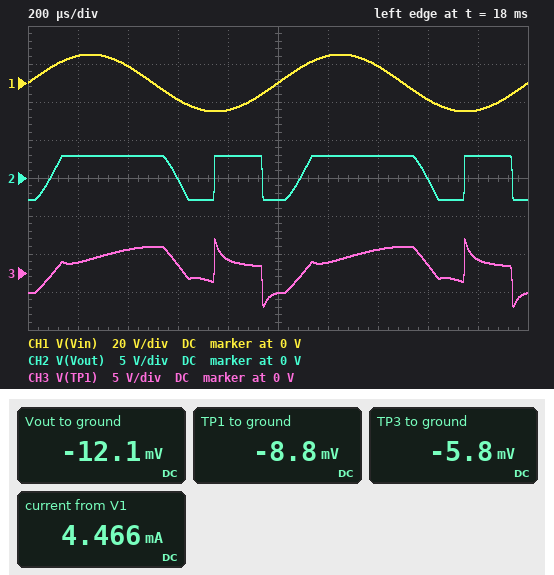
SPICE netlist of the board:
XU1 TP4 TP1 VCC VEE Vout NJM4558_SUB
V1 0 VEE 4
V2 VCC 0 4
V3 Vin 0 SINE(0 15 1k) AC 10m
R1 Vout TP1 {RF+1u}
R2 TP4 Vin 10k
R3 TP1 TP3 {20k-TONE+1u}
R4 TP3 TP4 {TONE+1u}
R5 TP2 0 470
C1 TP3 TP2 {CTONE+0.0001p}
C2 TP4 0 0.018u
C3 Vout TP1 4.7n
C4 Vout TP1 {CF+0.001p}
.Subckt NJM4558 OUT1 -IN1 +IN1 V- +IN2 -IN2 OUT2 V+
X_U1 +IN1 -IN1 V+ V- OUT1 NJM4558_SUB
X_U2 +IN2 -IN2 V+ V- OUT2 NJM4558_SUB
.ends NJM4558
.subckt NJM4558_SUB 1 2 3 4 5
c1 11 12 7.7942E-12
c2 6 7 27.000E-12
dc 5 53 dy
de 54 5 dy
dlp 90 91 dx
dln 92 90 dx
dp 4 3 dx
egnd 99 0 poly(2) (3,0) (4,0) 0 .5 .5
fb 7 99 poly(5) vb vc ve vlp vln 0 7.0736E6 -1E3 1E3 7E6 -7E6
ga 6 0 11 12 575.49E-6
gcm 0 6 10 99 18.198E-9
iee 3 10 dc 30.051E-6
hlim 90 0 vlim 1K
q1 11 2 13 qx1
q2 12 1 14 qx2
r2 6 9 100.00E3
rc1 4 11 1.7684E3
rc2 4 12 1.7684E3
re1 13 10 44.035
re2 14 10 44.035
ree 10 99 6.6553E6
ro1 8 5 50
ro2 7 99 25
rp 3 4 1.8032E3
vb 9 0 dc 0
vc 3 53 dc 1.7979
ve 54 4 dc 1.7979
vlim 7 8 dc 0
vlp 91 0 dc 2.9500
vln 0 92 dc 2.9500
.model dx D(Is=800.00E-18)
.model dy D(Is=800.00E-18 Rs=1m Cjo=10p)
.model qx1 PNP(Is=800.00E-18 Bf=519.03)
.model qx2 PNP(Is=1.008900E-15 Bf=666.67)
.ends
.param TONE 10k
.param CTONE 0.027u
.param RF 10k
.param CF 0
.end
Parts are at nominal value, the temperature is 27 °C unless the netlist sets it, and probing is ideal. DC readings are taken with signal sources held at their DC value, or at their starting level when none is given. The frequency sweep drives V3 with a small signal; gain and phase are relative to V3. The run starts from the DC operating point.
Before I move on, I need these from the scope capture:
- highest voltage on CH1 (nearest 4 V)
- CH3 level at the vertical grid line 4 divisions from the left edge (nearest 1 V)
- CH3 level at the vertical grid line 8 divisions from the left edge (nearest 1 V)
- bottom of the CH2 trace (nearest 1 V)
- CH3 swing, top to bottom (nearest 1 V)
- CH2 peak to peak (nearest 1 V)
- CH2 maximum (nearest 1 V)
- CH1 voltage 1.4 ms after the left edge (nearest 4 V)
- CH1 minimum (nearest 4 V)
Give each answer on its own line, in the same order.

16 V
2 V
1 V
-3 V
9 V
6 V
3 V
8 V
-16 V
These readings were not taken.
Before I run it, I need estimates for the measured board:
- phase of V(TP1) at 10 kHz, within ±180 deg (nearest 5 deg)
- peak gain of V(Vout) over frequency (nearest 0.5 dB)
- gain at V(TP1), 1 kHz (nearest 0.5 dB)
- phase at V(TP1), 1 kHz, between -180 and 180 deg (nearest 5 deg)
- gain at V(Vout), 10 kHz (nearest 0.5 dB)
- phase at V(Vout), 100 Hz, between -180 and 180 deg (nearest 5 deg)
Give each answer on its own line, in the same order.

-80 deg
0 dB
-6.5 dB
-50 deg
-20.0 dB
-5 deg
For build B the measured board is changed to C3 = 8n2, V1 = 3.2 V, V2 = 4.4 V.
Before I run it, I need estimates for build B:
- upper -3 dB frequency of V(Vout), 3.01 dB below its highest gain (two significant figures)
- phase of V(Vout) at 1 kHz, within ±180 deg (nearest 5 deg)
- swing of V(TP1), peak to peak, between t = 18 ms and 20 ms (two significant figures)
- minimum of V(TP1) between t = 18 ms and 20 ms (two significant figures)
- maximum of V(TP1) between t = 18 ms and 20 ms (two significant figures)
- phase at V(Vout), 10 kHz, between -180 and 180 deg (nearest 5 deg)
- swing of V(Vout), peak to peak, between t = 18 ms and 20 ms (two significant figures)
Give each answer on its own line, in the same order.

1.0 kHz
-40 deg
8.7 V
-3.7 V
5.0 V
-90 deg
5.5 V
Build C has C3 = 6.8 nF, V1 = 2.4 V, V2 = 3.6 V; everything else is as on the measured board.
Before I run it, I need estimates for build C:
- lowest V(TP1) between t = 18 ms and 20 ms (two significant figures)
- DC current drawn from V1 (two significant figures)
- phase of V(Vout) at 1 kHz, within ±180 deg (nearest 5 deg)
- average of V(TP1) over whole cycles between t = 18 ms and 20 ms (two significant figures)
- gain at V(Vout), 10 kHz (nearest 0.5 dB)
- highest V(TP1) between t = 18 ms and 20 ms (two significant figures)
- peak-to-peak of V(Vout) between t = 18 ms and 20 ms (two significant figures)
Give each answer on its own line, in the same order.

-2.8 V
3.4 mA
-40 deg
1.5 V
-20.5 dB
4.0 V
3.9 V
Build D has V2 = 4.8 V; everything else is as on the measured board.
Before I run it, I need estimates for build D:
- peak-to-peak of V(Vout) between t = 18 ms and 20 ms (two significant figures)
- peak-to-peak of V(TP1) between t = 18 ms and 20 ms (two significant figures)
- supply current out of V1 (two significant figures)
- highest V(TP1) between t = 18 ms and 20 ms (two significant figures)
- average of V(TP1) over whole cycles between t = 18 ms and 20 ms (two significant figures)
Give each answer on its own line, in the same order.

6.7 V
9.8 V
4.9 mA
5.3 V
1.3 V
